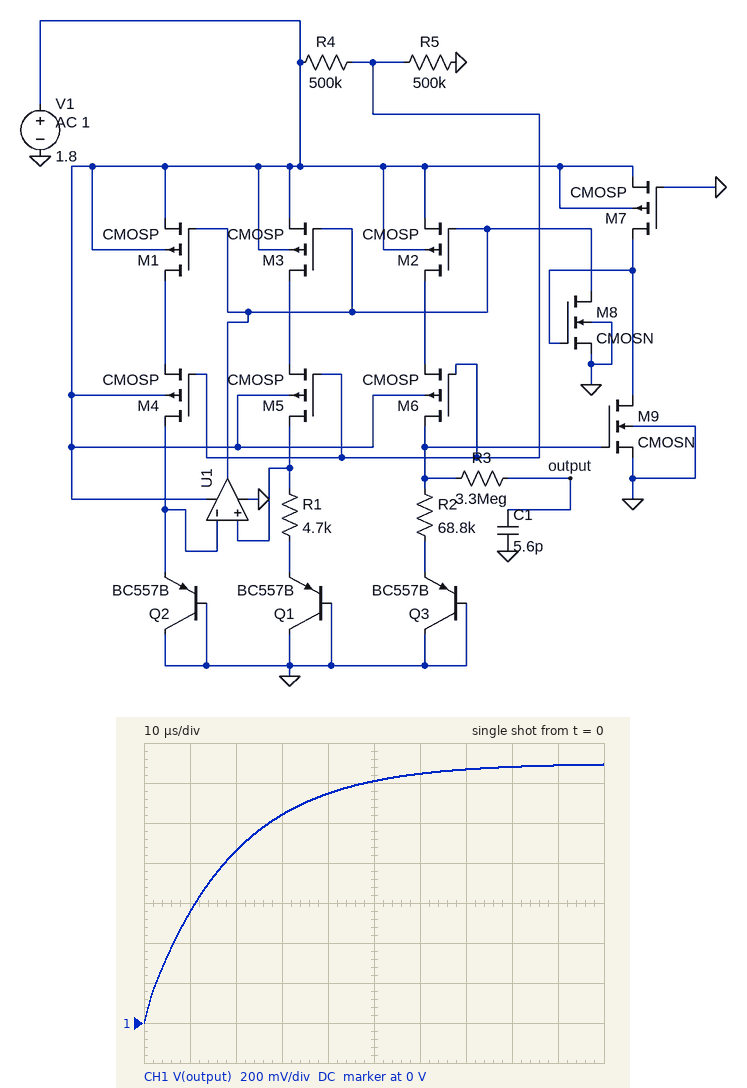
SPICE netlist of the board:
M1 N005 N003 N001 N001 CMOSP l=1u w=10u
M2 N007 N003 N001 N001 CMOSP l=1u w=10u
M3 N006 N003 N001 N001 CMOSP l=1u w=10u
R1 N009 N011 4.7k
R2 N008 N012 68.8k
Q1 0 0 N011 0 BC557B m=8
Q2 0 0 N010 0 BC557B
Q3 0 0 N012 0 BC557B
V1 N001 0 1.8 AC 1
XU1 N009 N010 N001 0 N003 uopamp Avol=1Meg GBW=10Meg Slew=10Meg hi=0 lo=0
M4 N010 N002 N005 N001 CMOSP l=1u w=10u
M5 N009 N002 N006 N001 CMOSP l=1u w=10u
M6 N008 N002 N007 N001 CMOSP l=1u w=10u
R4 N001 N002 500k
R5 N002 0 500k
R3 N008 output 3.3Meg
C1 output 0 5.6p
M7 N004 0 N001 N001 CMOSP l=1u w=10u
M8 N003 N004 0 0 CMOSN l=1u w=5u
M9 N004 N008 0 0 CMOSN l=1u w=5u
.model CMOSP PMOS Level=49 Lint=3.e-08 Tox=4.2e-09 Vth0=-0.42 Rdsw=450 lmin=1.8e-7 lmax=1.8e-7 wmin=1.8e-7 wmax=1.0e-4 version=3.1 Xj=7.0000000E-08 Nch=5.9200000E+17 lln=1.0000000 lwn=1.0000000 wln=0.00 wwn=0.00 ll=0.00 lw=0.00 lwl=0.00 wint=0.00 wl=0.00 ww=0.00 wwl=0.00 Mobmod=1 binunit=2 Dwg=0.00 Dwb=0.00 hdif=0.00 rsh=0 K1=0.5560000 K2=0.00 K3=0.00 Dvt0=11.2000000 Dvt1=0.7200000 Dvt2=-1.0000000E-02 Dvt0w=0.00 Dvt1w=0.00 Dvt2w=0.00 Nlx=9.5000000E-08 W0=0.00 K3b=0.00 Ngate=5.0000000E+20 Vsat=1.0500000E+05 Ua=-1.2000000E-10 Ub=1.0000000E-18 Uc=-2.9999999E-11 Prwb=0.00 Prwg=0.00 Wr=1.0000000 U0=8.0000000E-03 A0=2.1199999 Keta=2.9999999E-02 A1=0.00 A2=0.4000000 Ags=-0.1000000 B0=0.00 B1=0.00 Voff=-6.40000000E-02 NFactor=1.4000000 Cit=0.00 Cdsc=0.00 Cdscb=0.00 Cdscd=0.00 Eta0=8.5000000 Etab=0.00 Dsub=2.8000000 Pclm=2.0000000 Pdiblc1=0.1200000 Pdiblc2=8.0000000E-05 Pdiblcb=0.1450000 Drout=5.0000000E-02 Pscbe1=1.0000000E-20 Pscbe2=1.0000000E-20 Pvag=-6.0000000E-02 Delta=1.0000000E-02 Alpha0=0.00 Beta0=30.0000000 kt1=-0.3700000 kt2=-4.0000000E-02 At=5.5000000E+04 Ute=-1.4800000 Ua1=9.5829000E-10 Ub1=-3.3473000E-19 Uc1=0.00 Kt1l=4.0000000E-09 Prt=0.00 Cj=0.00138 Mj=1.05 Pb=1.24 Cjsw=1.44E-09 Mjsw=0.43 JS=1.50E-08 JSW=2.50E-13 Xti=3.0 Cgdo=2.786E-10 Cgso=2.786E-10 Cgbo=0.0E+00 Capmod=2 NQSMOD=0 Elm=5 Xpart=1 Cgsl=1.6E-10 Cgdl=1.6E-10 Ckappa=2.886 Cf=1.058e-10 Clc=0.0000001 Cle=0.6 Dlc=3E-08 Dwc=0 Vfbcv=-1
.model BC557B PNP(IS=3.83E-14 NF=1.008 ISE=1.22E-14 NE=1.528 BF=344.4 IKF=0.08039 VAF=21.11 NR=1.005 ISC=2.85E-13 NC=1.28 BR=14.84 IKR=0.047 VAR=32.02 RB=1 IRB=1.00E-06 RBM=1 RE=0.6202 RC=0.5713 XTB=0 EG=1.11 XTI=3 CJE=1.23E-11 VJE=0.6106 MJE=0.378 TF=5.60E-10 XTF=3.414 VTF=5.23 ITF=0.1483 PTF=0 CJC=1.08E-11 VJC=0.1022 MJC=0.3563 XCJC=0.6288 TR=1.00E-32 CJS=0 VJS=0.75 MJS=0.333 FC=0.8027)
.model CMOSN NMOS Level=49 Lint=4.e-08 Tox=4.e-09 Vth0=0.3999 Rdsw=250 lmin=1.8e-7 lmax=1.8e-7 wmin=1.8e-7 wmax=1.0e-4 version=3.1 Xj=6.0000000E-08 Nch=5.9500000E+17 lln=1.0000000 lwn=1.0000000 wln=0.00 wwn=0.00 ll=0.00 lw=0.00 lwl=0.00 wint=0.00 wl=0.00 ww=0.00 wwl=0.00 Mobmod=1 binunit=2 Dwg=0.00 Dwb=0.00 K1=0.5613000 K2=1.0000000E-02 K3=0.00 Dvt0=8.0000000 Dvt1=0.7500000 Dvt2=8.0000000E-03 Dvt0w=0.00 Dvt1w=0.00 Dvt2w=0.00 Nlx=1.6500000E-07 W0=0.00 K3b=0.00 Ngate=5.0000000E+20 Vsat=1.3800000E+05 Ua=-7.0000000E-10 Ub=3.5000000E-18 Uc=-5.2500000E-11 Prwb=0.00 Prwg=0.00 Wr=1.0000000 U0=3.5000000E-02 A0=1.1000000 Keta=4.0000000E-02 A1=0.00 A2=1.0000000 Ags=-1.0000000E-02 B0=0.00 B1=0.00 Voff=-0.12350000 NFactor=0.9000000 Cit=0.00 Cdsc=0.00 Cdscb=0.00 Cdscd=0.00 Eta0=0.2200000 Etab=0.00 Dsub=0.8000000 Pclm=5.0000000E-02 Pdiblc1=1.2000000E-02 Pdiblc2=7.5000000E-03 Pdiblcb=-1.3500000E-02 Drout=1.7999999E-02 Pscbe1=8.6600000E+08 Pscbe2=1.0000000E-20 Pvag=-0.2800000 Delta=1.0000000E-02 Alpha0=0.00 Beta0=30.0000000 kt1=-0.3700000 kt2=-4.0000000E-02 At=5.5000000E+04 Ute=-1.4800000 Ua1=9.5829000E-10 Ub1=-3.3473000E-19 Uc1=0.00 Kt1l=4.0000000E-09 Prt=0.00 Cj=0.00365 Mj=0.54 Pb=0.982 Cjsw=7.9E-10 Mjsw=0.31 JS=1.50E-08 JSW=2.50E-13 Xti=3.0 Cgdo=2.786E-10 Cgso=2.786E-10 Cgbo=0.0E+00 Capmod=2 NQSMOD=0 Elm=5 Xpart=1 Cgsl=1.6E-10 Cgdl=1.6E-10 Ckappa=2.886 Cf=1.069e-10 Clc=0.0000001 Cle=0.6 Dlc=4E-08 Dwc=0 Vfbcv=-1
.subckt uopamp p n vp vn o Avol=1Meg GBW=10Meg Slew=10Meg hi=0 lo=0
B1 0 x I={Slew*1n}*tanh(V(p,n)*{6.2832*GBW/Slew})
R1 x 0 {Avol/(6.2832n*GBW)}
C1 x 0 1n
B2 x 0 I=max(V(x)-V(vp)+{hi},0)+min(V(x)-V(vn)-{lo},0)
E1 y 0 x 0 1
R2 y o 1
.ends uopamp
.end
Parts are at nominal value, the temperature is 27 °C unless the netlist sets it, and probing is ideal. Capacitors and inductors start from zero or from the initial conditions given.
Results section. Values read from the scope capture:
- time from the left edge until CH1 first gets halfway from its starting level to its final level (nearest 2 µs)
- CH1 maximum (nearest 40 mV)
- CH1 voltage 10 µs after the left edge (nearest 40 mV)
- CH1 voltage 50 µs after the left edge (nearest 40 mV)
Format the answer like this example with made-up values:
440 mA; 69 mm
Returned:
12 µs; 1.28 V; 560 mV; 1.20 V
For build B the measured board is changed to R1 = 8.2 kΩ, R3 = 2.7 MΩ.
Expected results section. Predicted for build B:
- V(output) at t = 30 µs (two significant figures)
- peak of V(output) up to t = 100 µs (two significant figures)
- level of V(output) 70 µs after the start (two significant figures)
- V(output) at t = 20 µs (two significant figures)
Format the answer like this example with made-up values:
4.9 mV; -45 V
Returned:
830 mV; 950 mV; 940 mV; 710 mV
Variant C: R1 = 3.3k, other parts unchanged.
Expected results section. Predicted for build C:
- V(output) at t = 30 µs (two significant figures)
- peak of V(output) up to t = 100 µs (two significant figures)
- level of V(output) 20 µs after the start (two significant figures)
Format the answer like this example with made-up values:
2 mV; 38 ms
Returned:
1.2 V; 1.5 V; 1.0 V
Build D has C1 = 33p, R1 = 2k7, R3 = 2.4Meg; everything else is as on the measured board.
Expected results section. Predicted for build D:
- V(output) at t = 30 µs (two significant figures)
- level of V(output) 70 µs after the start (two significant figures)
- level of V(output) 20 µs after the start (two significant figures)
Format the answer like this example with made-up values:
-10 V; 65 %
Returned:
500 mV; 940 mV; 360 mV
